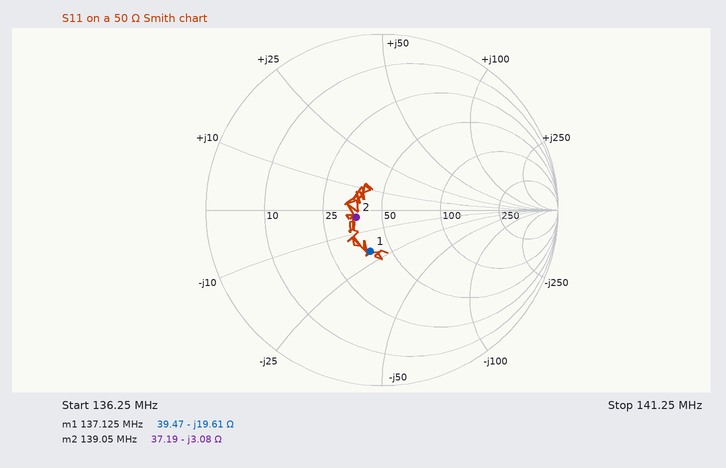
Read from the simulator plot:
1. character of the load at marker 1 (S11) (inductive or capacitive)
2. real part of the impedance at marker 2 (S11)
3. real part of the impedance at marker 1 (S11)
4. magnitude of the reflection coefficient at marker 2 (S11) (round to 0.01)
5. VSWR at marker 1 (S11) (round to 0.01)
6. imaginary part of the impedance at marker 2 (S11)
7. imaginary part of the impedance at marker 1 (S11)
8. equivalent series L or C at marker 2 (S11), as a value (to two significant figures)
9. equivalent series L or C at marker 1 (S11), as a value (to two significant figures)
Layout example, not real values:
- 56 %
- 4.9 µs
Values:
- capacitive
- 37.19 Ω
- 39.47 Ω
- 0.15
- 1.64
- -3.08 Ω
- -19.61 Ω
- 370 pF
- 59 pF
